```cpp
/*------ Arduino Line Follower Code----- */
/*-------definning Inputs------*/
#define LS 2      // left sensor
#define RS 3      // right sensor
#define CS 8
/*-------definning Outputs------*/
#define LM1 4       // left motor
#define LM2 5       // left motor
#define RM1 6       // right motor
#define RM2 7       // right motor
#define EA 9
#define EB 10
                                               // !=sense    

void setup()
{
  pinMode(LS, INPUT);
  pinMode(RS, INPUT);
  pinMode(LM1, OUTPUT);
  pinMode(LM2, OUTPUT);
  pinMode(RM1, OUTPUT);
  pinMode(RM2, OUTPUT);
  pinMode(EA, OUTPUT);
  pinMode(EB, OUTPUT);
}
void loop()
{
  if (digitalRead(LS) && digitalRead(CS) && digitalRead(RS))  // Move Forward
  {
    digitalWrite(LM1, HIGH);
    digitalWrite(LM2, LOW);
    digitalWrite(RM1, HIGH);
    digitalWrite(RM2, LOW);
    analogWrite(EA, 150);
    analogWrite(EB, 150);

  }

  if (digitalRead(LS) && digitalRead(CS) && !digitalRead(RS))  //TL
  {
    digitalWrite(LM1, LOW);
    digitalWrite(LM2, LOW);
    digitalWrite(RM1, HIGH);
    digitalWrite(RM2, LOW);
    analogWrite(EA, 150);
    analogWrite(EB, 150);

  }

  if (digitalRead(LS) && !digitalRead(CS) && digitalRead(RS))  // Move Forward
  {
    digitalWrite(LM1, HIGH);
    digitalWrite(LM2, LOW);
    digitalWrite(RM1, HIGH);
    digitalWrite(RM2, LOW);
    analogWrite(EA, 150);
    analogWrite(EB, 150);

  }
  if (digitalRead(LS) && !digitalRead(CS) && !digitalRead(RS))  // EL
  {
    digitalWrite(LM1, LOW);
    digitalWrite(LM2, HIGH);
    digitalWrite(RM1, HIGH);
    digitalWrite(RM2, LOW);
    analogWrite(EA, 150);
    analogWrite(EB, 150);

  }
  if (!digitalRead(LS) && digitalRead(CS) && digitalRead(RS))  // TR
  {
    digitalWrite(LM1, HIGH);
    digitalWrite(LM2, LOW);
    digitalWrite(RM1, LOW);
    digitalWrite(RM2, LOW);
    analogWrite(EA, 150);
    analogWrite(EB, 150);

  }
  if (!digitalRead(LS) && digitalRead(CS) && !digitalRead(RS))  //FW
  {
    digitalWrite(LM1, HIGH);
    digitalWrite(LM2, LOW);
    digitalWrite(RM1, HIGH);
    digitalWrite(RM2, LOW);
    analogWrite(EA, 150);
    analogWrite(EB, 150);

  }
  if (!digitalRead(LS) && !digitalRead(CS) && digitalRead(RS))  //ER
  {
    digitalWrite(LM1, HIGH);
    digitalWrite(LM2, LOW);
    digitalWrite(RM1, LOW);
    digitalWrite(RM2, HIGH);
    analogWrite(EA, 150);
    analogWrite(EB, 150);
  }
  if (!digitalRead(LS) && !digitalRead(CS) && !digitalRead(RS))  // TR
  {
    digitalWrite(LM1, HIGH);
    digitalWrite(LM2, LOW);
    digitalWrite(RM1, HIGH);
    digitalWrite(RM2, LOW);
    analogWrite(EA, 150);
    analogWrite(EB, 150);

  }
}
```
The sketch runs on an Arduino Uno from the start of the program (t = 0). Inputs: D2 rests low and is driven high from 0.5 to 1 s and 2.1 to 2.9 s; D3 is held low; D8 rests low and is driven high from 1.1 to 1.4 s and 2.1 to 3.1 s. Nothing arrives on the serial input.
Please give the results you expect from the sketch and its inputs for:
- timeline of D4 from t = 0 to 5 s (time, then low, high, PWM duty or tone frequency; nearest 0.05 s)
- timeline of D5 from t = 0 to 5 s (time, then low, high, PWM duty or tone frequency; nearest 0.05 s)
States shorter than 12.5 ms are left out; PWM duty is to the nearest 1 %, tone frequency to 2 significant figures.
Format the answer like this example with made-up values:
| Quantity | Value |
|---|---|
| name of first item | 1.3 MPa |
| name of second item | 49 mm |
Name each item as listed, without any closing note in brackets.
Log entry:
| Quantity | Value |
|---|---|
| timeline of D4 from t = 0 to 5 s | 0 s high; 0.5 s low; 1 s high; 2.1 s low; 2.9 s high |
| timeline of D5 from t = 0 to 5 s | 0 s low; 0.5 s high; 1 s low |
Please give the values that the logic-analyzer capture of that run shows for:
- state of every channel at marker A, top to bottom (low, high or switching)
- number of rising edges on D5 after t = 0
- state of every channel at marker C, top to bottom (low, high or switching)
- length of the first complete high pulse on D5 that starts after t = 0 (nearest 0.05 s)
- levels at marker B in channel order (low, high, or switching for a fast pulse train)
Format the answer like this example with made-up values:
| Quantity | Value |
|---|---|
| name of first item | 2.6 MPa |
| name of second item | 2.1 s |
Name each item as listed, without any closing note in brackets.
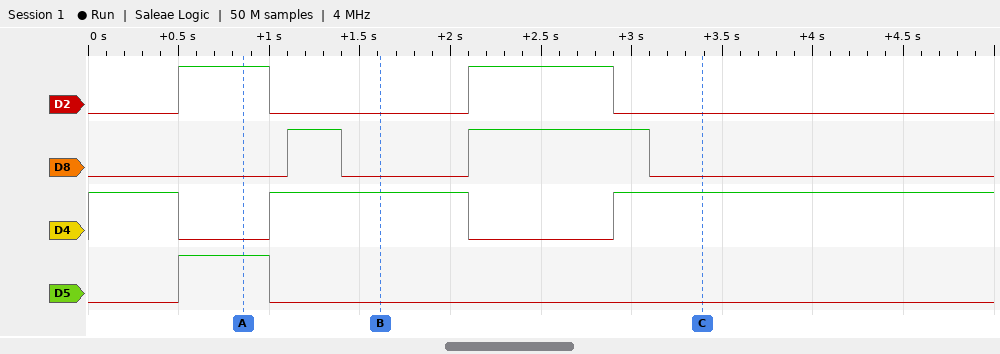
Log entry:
| Quantity | Value |
|---|---|
| state of every channel at marker A, top to bottom | D2 high, D8 low, D4 low, D5 high |
| number of rising edges on D5 after t = 0 | 1 |
| state of every channel at marker C, top to bottom | D2 low, D8 low, D4 high, D5 low |
| length of the first complete high pulse on D5 that starts after t = 0 | 0.50 s |
| levels at marker B in channel order | D2 low, D8 low, D4 high, D5 low |
